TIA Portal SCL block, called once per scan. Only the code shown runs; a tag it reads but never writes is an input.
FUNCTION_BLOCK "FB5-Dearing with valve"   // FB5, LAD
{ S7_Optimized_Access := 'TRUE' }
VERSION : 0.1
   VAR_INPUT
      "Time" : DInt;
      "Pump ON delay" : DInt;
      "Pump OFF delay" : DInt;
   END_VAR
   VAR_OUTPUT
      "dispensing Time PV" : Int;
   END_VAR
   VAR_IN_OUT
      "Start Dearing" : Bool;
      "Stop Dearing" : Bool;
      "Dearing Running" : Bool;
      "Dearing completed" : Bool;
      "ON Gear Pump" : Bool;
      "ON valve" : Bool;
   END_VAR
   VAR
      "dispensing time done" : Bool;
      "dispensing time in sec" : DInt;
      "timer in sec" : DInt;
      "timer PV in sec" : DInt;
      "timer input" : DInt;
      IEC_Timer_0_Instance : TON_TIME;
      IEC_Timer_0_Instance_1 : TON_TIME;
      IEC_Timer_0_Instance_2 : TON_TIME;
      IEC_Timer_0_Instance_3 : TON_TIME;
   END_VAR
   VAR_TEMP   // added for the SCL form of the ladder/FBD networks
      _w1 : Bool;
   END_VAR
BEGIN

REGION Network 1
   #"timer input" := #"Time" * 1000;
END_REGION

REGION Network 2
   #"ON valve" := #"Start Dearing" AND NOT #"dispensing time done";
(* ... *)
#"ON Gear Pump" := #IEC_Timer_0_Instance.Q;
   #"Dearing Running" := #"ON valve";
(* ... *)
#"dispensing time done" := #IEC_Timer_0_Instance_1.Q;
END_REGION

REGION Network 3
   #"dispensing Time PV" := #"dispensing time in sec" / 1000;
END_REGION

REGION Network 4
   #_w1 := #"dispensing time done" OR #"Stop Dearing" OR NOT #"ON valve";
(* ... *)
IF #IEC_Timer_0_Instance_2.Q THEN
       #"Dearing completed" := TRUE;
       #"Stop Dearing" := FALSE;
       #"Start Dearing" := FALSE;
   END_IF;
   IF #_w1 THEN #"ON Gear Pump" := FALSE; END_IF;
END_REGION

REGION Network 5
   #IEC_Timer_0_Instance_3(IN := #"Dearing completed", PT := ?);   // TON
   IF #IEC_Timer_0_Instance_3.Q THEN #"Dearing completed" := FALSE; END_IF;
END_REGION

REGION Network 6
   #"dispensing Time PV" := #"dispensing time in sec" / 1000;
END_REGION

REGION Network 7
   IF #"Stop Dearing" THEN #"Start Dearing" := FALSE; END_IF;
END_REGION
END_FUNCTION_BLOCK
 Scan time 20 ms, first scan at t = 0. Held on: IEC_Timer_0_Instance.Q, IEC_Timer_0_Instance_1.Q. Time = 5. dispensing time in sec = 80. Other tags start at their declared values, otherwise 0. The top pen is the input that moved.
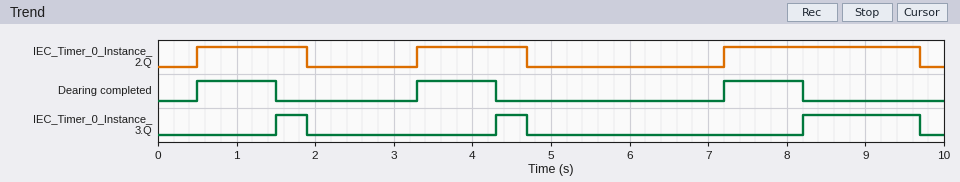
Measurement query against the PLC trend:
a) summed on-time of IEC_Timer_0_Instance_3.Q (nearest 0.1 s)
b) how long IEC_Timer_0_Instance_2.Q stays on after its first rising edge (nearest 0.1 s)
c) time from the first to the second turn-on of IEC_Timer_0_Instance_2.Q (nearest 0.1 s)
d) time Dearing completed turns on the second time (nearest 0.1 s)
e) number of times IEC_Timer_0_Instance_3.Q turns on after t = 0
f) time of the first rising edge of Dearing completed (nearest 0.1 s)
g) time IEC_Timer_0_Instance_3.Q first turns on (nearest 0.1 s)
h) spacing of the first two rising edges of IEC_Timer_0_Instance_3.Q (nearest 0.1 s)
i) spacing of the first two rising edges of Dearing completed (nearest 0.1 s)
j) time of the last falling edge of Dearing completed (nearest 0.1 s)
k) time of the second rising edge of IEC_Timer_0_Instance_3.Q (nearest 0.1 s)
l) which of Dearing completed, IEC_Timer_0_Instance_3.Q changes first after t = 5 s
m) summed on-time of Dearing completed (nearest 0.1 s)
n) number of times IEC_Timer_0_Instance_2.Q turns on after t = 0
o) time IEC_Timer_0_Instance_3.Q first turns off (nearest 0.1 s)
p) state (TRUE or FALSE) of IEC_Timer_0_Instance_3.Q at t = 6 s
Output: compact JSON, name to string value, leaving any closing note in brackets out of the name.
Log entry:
{"summed on-time of IEC_Timer_0_Instance_3.Q": "2.3 s", "how long IEC_Timer_0_Instance_2.Q stays on after its first rising edge": "1.4 s", "time from the first to the second turn-on of IEC_Timer_0_Instance_2.Q": "2.8 s", "time Dearing completed turns on the second time": "3.3 s", "number of times IEC_Timer_0_Instance_3.Q turns on after t = 0": "3", "time of the first rising edge of Dearing completed": "0.5 s", "time IEC_Timer_0_Instance_3.Q first turns on": "1.5 s", "spacing of the first two rising edges of IEC_Timer_0_Instance_3.Q": "2.8 s", "spacing of the first two rising edges of Dearing completed": "2.8 s", "time of the last falling edge of Dearing completed": "8.2 s", "time of the second rising edge of IEC_Timer_0_Instance_3.Q": "4.3 s", "which of Dearing completed, IEC_Timer_0_Instance_3.Q changes first after t = 5 s": "Dearing completed", "summed on-time of Dearing completed": "3.0 s", "number of times IEC_Timer_0_Instance_2.Q turns on after t = 0": "3", "time IEC_Timer_0_Instance_3.Q first turns off": "1.9 s", "state (TRUE or FALSE) of IEC_Timer_0_Instance_3.Q at t = 6 s": "FALSE"}
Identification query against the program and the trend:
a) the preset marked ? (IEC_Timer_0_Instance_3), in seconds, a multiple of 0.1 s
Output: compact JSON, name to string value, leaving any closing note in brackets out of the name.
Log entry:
{"the preset marked ? (IEC_Timer_0_Instance_3), in seconds, a multiple of 0.1 s": "1.0 s"}
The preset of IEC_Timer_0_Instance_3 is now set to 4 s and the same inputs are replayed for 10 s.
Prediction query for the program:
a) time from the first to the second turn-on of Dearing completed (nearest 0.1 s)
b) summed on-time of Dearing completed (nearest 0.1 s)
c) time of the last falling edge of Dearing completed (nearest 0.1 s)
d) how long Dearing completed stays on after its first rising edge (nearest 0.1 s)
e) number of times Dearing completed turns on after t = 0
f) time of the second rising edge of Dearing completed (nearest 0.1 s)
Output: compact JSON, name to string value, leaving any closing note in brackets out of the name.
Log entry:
{"time from the first to the second turn-on of Dearing completed": "6.7 s", "summed on-time of Dearing completed": "6.8 s", "time of the last falling edge of Dearing completed": "4.5 s", "how long Dearing completed stays on after its first rising edge": "4.0 s", "number of times Dearing completed turns on after t = 0": "2", "time of the second rising edge of Dearing completed": "7.2 s"}
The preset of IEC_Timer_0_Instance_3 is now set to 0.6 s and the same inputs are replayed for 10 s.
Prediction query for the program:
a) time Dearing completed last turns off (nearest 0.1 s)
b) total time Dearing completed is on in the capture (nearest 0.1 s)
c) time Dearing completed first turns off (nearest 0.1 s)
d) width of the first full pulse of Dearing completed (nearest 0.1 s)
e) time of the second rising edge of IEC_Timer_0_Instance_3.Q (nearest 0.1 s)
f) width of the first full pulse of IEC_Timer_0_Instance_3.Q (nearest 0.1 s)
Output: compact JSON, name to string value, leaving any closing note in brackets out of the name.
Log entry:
{"time Dearing completed last turns off": "7.8 s", "total time Dearing completed is on in the capture": "1.8 s", "time Dearing completed first turns off": "1.1 s", "width of the first full pulse of Dearing completed": "0.6 s", "time of the second rising edge of IEC_Timer_0_Instance_3.Q": "3.9 s", "width of the first full pulse of IEC_Timer_0_Instance_3.Q": "0.8 s"}
